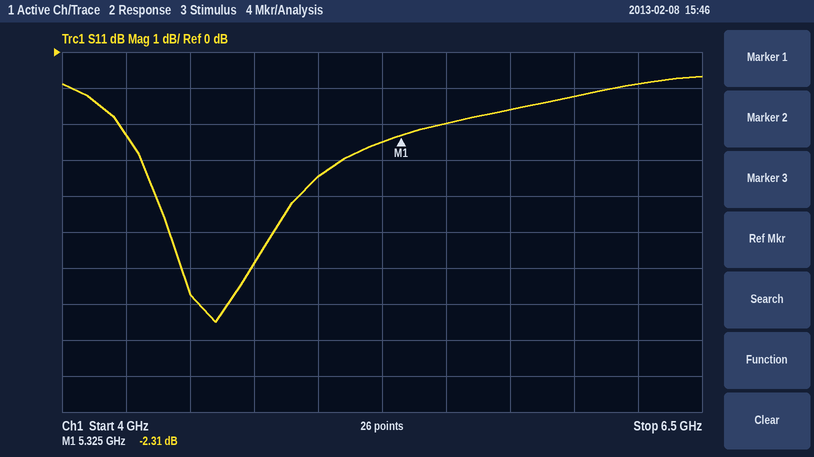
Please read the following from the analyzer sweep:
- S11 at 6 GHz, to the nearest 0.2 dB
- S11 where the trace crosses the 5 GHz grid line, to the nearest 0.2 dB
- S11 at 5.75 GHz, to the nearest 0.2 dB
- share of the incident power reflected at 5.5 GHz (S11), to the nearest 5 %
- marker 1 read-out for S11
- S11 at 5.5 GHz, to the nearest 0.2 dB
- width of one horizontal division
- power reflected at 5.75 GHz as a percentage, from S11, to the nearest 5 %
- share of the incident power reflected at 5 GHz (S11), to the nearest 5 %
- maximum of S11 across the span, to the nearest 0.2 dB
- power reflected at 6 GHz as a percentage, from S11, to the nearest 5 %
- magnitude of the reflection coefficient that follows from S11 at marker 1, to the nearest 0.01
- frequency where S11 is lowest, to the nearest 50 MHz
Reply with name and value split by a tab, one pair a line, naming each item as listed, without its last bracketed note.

S11 at 6 GHz, to the nearest 0.2 dB	-1.2 dB
S11 where the trace crosses the 5 GHz grid line, to the nearest 0.2 dB	-3.4 dB
S11 at 5.75 GHz, to the nearest 0.2 dB	-1.6 dB
share of the incident power reflected at 5.5 GHz (S11), to the nearest 5 %	65 %
marker 1 read-out for S11	-2.31 dB
S11 at 5.5 GHz, to the nearest 0.2 dB	-2.0 dB
width of one horizontal division	250 MHz
power reflected at 5.75 GHz as a percentage, from S11, to the nearest 5 %	70 %
share of the incident power reflected at 5 GHz (S11), to the nearest 5 %	45 %
maximum of S11 across the span, to the nearest 0.2 dB	-0.6 dB
power reflected at 6 GHz as a percentage, from S11, to the nearest 5 %	75 %
magnitude of the reflection coefficient that follows from S11 at marker 1, to the nearest 0.01	0.77
frequency where S11 is lowest, to the nearest 50 MHz	4.60 GHz
